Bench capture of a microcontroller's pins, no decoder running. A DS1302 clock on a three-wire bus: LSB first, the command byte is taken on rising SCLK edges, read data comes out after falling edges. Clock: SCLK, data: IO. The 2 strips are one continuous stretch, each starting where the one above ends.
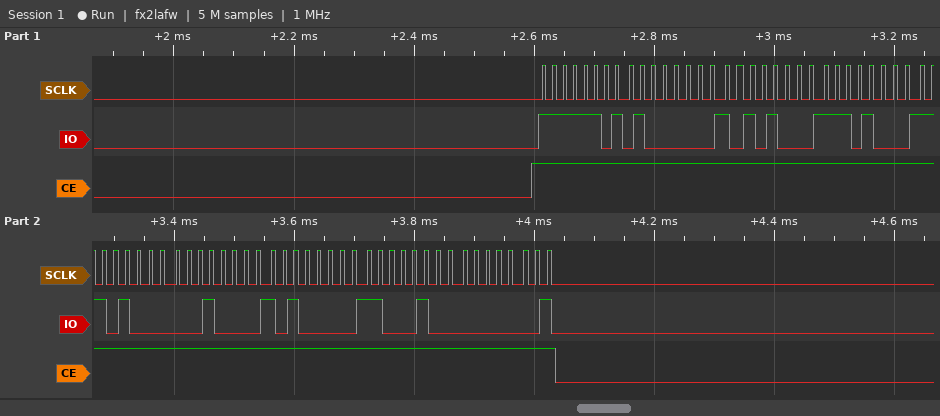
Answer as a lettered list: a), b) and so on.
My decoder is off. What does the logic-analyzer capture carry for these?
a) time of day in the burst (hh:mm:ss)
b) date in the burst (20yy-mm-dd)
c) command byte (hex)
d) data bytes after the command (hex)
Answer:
a) 17:15:02
b) 2023-08-17
c) 0xBF
d) 02 15 17 17 08 05 23 80
